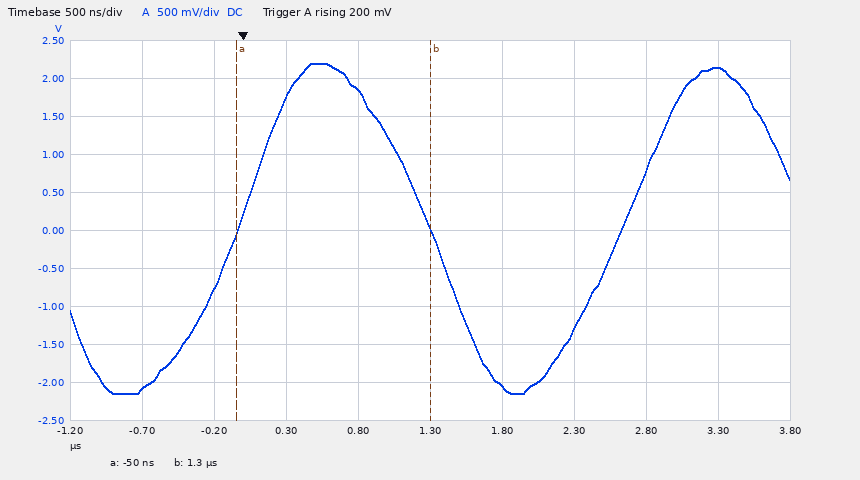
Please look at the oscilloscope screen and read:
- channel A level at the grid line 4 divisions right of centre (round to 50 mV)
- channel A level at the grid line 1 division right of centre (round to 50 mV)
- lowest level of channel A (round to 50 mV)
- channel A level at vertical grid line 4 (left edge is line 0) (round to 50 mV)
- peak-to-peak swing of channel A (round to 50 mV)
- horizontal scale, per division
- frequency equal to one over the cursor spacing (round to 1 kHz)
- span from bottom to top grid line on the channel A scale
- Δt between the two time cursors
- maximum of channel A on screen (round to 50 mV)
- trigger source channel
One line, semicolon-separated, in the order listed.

2.15 V; -2.05 V; -2.15 V; 1.85 V; 4.35 V; 500 ns; 741 kHz; 5 V; 1.35 µs; 2.20 V; channel A
